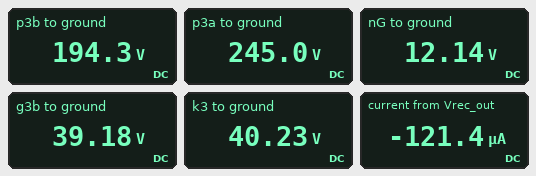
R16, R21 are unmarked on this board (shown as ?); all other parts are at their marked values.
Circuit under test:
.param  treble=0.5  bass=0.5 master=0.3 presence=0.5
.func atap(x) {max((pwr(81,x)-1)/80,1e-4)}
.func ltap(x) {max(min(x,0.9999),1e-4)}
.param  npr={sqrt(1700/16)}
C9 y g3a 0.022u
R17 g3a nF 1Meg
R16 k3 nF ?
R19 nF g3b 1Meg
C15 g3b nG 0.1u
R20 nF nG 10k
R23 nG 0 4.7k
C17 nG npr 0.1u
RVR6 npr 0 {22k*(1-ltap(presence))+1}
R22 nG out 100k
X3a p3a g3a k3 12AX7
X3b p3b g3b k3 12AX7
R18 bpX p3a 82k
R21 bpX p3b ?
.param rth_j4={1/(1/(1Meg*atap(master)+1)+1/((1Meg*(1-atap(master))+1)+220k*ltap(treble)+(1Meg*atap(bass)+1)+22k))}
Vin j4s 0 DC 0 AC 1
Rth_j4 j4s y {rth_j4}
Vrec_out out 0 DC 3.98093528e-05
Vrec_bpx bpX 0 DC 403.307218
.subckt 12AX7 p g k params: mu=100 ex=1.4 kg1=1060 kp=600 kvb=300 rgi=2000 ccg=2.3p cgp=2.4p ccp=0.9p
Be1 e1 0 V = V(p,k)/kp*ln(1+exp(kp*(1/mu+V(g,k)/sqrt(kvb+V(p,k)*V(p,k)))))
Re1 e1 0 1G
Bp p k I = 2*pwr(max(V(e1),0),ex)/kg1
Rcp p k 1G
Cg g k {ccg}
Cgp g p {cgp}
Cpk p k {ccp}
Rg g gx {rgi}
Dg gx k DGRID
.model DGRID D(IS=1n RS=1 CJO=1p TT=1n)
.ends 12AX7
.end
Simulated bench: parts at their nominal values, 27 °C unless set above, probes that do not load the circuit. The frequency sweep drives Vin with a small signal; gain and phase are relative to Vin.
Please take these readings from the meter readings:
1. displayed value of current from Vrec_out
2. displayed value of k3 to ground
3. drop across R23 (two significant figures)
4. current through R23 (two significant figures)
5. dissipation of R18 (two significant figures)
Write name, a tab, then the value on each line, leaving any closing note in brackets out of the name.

displayed value of current from Vrec_out	-121.4 µA
displayed value of k3 to ground	40.23 V
drop across R23	12 V
current through R23	2.6 mA
dissipation of R18	310 mW
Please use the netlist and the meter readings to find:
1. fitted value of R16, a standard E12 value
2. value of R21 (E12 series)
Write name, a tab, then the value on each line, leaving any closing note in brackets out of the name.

fitted value of R16, a standard E12 value	390 Ω
value of R21	270 kΩ
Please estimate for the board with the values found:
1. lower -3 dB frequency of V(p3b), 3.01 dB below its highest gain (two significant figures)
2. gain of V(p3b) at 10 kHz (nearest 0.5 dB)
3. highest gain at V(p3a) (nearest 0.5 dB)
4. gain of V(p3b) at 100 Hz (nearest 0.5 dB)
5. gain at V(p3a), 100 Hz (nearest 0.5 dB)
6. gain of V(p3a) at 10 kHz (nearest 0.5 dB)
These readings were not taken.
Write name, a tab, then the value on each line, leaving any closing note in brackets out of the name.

lower -3 dB frequency of V(p3b), 3.01 dB below its highest gain	3.4 Hz
gain of V(p3b) at 10 kHz	32.5 dB
highest gain at V(p3a)	25.0 dB
gain of V(p3b) at 100 Hz	32.5 dB
gain at V(p3a), 100 Hz	24.5 dB
gain of V(p3a) at 10 kHz	25.0 dB
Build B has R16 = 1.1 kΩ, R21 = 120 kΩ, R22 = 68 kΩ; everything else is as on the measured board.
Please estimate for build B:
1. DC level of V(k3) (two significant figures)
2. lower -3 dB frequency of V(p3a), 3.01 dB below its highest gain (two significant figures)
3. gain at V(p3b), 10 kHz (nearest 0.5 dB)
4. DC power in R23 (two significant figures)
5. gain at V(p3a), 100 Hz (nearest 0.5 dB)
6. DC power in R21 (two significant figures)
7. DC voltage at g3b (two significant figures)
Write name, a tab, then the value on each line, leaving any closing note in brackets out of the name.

DC level of V(k3)	31 V
lower -3 dB frequency of V(p3a), 3.01 dB below its highest gain	4.2 Hz
gain at V(p3b), 10 kHz	28.5 dB
DC power in R23	17 mW
gain at V(p3a), 100 Hz	26.5 dB
DC power in R21	94 mW
DC voltage at g3b	29 V
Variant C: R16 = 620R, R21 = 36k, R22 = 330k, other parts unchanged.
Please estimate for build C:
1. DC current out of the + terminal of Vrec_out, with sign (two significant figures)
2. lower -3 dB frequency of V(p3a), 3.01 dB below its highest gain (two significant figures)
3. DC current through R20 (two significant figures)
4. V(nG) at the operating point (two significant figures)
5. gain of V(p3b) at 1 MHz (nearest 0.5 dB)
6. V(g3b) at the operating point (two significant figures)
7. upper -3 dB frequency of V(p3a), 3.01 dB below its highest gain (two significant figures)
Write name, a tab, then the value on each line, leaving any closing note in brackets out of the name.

DC current out of the + terminal of Vrec_out, with sign	-44 µA
lower -3 dB frequency of V(p3a), 3.01 dB below its highest gain	5.1 Hz
DC current through R20	3.1 mA
V(nG) at the operating point	14 V
gain of V(p3b) at 1 MHz	0 dB
V(g3b) at the operating point	46 V
upper -3 dB frequency of V(p3a), 3.01 dB below its highest gain	53 kHz
